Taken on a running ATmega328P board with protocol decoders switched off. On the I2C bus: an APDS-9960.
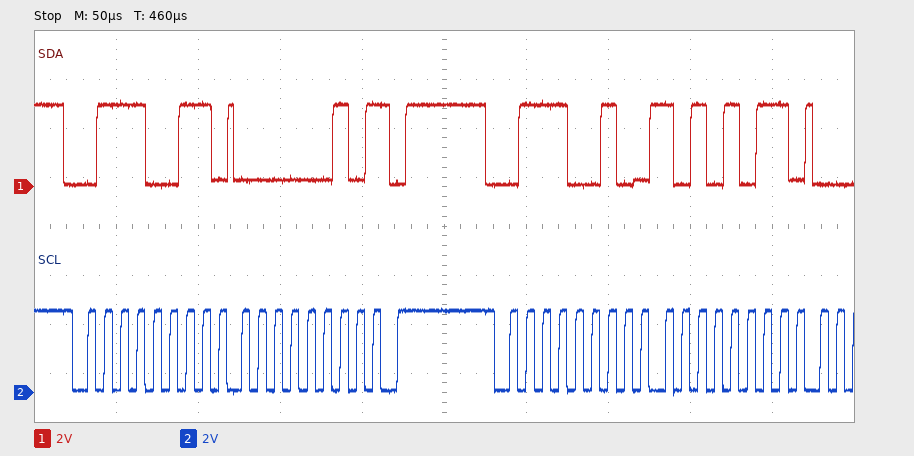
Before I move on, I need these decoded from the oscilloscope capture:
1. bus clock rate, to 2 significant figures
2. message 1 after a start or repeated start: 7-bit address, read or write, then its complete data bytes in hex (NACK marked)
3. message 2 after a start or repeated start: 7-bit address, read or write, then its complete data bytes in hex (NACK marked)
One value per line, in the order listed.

100 kHz
0x39 read: 02 NACK
0x39 write: AB
